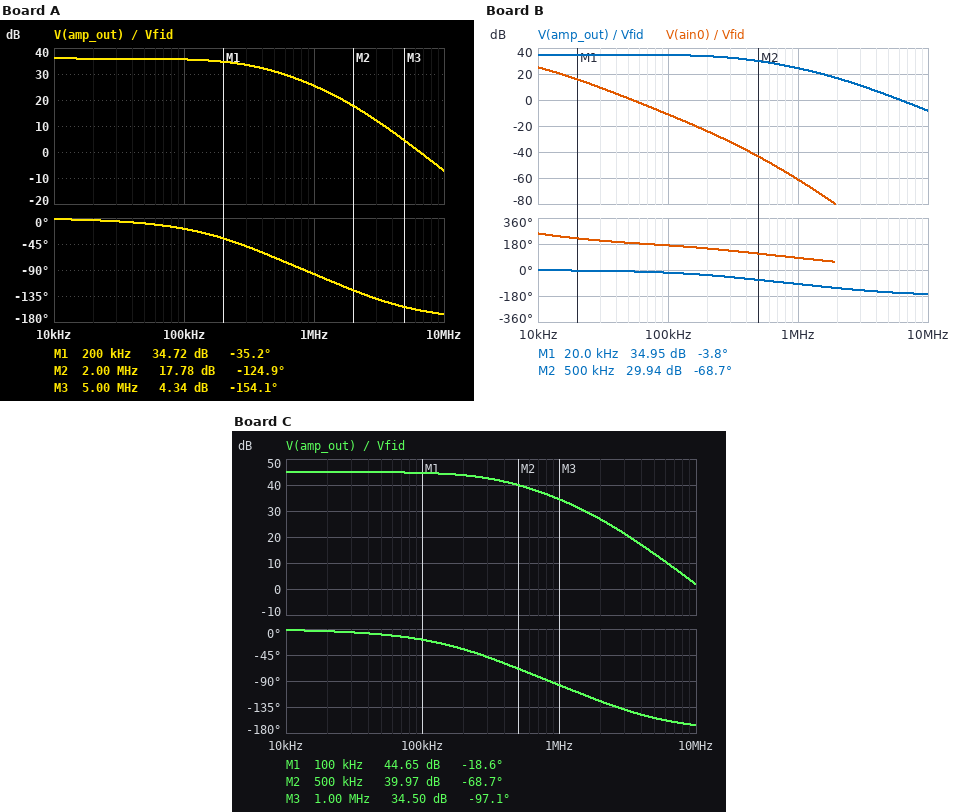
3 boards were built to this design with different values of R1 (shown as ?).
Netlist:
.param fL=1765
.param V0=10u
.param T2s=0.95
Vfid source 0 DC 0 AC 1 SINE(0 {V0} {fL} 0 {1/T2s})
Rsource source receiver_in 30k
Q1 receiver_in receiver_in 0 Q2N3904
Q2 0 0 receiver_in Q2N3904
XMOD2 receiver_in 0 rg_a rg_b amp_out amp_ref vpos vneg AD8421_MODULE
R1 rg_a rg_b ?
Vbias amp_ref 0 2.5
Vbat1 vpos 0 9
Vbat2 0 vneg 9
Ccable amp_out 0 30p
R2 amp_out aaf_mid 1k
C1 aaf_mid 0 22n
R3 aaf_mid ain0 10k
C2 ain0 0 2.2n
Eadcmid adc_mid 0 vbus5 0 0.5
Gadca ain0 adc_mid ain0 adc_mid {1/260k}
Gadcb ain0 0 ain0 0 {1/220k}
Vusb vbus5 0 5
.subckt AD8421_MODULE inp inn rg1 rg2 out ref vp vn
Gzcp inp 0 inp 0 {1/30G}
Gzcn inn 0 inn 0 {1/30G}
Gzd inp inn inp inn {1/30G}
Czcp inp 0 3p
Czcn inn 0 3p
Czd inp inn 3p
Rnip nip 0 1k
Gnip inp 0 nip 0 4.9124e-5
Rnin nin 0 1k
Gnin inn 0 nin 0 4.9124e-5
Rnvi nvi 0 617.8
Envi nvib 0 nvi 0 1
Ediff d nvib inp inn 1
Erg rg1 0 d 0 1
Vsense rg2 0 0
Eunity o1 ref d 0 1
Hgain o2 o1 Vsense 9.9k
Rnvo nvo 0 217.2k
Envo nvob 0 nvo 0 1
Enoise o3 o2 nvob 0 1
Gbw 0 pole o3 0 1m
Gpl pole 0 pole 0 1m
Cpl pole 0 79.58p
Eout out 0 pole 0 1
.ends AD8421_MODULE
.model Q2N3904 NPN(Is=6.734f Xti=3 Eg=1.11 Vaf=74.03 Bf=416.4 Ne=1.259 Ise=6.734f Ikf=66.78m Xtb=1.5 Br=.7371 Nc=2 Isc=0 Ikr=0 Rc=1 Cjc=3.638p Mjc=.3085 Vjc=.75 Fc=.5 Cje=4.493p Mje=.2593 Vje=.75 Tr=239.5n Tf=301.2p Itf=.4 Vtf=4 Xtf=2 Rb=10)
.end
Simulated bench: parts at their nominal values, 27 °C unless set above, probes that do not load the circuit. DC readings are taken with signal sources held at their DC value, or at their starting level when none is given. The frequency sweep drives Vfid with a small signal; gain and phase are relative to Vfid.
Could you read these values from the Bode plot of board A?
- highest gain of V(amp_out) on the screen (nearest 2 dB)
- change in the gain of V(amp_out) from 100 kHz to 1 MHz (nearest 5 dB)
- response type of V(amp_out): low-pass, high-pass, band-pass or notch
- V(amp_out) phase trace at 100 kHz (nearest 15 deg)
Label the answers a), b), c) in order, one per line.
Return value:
a) 36 dB
b) -10 dB
c) low-pass
d) -15 deg
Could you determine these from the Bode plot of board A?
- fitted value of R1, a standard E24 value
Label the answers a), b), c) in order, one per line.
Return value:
a) 160 Ω
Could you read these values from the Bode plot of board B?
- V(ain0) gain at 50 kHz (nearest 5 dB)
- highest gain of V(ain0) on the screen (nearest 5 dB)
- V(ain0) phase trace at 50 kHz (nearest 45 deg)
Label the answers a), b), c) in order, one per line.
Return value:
a) 0 dB
b) 25 dB
c) 180 deg
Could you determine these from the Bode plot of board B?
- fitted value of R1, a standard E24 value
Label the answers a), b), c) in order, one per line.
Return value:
a) 180 Ω
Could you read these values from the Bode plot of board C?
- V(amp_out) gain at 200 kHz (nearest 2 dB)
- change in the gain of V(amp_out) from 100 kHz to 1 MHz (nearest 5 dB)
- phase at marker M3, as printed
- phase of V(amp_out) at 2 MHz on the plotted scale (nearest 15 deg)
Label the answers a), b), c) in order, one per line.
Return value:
a) 44 dB
b) -10 dB
c) -97.1 deg
d) -120 deg
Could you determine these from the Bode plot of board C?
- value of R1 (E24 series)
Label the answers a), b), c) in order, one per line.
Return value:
a) 56 Ω
